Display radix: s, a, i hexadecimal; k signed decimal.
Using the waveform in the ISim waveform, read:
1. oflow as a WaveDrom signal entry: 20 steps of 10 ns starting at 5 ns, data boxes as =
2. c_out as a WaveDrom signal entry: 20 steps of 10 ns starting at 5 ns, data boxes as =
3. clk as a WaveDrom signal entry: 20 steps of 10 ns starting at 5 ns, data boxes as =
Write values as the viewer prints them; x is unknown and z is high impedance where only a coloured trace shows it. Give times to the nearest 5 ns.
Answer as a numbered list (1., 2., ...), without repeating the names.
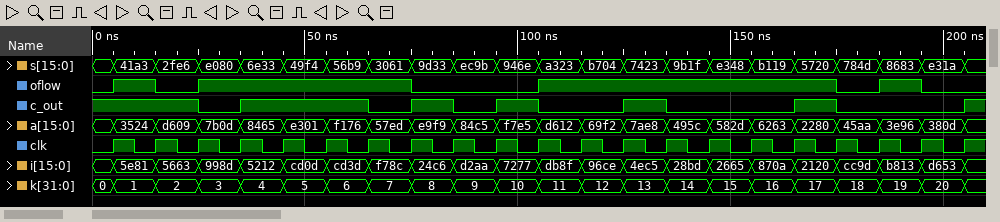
1. {name: 'oflow', wave: '101....0..1......010'}
2. {name: 'c_out', wave: '1.01..01010.10..10..'}
3. {name: 'clk', wave: 'p...................'}
